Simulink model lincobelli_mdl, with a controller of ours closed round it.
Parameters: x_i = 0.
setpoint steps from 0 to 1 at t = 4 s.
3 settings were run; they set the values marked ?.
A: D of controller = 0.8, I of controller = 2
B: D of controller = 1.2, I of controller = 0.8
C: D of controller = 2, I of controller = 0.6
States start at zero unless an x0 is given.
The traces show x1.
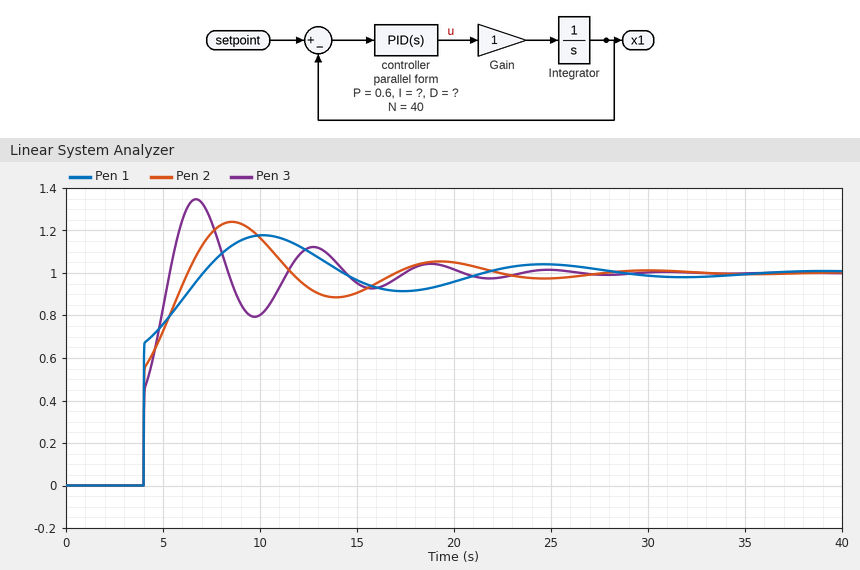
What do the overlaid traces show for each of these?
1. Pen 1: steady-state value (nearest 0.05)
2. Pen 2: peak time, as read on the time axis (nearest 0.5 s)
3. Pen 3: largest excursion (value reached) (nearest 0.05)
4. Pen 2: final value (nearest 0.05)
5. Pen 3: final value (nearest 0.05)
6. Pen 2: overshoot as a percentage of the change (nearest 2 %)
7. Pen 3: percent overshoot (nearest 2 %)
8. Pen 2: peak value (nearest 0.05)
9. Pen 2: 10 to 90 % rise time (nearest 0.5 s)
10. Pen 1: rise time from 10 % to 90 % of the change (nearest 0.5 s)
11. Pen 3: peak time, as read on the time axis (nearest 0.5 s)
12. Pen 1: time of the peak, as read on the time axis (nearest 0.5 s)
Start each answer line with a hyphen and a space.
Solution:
- 1.00
- 8.5 s
- 1.35
- 1.00
- 1.00
- 24 %
- 34 %
- 1.25
- 2.0 s
- 2.0 s
- 6.5 s
- 10.0 s
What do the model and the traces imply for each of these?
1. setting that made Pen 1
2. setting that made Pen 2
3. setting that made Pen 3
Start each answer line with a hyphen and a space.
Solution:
- C
- B
- A
